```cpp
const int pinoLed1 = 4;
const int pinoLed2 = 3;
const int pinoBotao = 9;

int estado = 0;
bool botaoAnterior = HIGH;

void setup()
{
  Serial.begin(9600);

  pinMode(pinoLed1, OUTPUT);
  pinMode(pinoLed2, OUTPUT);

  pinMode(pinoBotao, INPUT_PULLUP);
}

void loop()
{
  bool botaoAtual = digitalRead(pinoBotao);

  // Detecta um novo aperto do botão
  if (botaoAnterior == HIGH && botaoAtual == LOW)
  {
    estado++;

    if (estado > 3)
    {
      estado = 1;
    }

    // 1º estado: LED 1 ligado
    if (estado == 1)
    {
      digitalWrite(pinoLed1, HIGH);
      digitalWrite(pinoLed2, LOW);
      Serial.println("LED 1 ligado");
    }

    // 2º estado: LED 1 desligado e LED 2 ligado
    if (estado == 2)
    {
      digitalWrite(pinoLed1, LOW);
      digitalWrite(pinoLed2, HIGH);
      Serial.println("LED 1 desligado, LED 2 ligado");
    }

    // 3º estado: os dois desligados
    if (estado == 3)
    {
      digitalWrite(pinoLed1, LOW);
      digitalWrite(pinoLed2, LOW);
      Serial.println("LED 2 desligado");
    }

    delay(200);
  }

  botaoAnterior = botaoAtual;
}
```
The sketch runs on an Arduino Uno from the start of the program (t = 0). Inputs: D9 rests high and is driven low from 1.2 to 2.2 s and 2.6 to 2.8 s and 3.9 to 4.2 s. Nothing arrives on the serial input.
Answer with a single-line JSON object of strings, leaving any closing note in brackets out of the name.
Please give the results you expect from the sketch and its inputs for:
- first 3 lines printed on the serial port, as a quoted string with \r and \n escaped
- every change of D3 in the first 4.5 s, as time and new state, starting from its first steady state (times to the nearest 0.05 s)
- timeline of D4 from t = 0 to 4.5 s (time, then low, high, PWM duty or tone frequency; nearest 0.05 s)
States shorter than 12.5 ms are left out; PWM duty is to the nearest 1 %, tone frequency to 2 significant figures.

{"first 3 lines printed on the serial port, as a quoted string with \\r and \\n escaped": "\"LED 1 ligado\\r\\nLED 1 desligado, LED 2 ligado\\r\\nLED 2 desligado\\r\\n\"", "every change of D3 in the first 4.5 s, as time and new state, starting from its first steady state": "0 s low; 2.6 s high; 3.9 s low", "timeline of D4 from t = 0 to 4.5 s": "0 s low; 1.2 s high; 2.6 s low"}
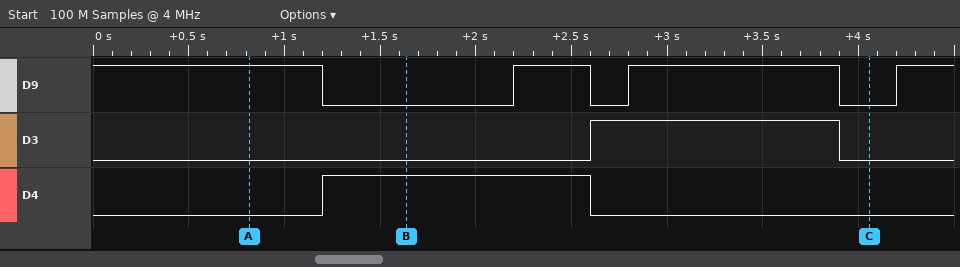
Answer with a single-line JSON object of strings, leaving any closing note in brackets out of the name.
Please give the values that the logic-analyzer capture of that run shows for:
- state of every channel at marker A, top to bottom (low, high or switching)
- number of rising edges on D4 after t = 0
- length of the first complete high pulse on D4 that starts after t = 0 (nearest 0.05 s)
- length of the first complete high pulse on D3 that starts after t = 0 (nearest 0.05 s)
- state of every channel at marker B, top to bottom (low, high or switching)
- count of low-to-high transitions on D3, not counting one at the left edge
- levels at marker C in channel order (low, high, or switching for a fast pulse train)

{"state of every channel at marker A, top to bottom": "D9 high, D3 low, D4 low", "number of rising edges on D4 after t = 0": "1", "length of the first complete high pulse on D4 that starts after t = 0": "1.40 s", "length of the first complete high pulse on D3 that starts after t = 0": "1.30 s", "state of every channel at marker B, top to bottom": "D9 low, D3 low, D4 high", "count of low-to-high transitions on D3, not counting one at the left edge": "1", "levels at marker C in channel order": "D9 low, D3 low, D4 low"}
